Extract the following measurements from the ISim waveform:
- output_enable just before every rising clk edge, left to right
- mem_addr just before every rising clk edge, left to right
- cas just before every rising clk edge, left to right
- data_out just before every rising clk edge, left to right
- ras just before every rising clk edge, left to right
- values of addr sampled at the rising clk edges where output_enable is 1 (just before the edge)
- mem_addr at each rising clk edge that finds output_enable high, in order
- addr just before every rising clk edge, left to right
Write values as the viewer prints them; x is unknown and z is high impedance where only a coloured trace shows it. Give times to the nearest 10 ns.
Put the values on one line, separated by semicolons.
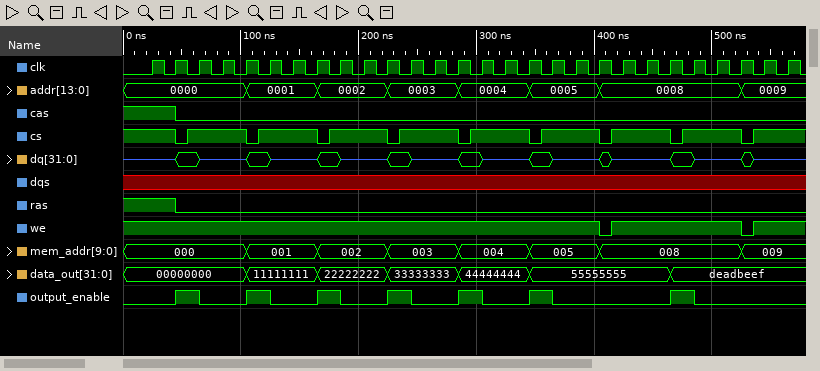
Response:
0 0 1 0 0 1 0 0 1 0 0 1 0 0 1 0 0 1 0 0 0 0 0 1 0 0 0 0; 000, 000, 000, 000, 000, 001, 001, 001, 002, 002, 002, 003, 003, 003, 004, 004, 004, 005, 005, 005, 008, 008, 008, 008, 008, 008, 009, 009; 1 1 0 0 0 0 0 0 0 0 0 0 0 0 0 0 0 0 0 0 0 0 0 0 0 0 0 0; 00000000, 00000000, 00000000, 00000000, 00000000, 11111111, 11111111, 11111111, 22222222, 22222222, 22222222, 33333333, 33333333, 33333333, 44444444, 44444444, 44444444, 55555555, 55555555, 55555555, 55555555, 55555555, 55555555, deadbeef, deadbeef, deadbeef, deadbeef, deadbeef; 1 1 0 0 0 0 0 0 0 0 0 0 0 0 0 0 0 0 0 0 0 0 0 0 0 0 0 0; 0000, 0001, 0002, 0003, 0004, 0005, 0008; 000, 001, 002, 003, 004, 005, 008; 0000, 0000, 0000, 0000, 0000, 0001, 0001, 0001, 0002, 0002, 0002, 0003, 0003, 0003, 0004, 0004, 0004, 0005, 0005, 0005, 0008, 0008, 0008, 0008, 0008, 0008, 0009, 0009
